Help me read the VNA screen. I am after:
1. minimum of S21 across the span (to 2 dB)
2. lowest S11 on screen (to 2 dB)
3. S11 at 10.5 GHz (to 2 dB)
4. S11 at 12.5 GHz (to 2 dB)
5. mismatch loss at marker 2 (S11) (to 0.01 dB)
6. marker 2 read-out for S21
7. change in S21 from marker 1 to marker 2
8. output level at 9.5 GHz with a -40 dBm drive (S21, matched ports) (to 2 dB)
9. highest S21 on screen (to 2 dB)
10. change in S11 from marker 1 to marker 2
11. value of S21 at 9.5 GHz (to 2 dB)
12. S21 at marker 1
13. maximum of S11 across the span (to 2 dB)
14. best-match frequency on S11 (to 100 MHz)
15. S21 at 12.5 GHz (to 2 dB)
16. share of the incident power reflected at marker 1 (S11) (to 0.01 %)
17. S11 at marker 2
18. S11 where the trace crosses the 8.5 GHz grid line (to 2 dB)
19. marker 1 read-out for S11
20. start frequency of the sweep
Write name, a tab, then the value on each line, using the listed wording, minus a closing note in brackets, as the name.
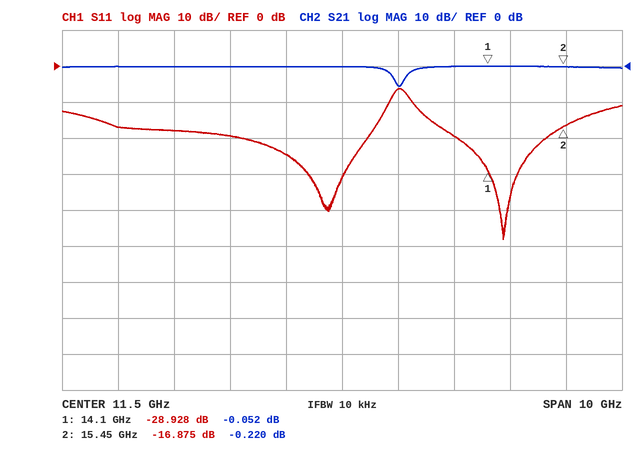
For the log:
minimum of S21 across the span	-6 dB
lowest S11 on screen	-48 dB
S11 at 10.5 GHz	-24 dB
S11 at 12.5 GHz	-6 dB
mismatch loss at marker 2 (S11)	0.09 dB
marker 2 read-out for S21	-0.220 dB
change in S21 from marker 1 to marker 2	-0.168 dB
output level at 9.5 GHz with a -40 dBm drive (S21, matched ports)	-40 dBm
highest S21 on screen	0 dB
change in S11 from marker 1 to marker 2	12.053 dB
value of S21 at 9.5 GHz	0 dB
S21 at marker 1	-0.052 dB
maximum of S11 across the span	-6 dB
best-match frequency on S11	14.4 GHz
S21 at 12.5 GHz	-6 dB
share of the incident power reflected at marker 1 (S11)	0.13 %
S11 at marker 2	-16.875 dB
S11 where the trace crosses the 8.5 GHz grid line	-18 dB
marker 1 read-out for S11	-28.928 dB
start frequency of the sweep	6.5 GHz
